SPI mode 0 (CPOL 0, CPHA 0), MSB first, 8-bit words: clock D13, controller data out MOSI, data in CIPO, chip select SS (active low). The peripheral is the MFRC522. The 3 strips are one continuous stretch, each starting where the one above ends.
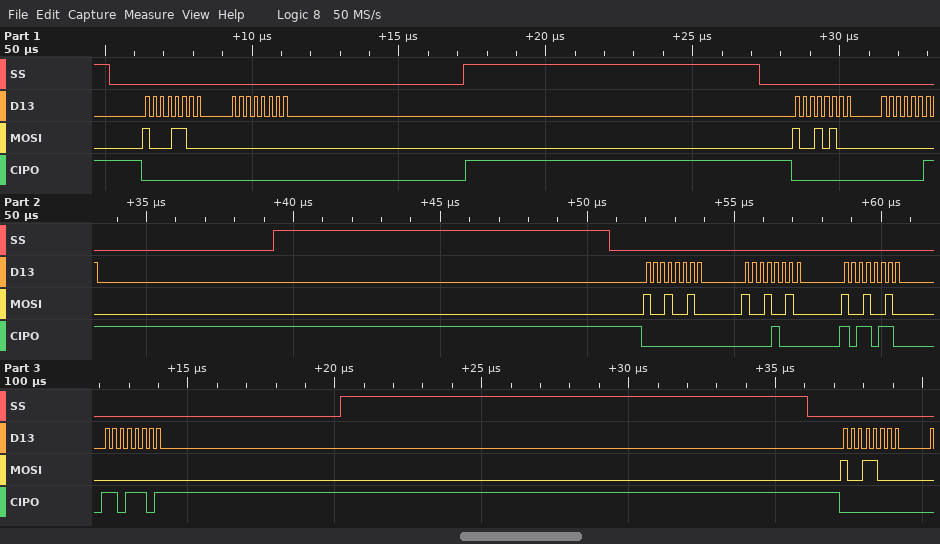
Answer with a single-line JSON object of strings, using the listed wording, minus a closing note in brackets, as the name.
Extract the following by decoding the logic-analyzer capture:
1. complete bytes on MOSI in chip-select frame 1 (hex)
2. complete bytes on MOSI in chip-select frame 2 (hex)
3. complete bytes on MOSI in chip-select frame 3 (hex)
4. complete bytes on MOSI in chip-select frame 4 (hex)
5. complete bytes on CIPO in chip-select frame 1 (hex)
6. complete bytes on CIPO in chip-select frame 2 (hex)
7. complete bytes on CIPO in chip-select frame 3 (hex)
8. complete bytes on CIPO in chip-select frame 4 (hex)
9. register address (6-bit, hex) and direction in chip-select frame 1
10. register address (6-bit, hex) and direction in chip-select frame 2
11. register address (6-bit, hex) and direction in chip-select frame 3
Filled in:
{"complete bytes on MOSI in chip-select frame 1": "0x8C 0x00", "complete bytes on MOSI in chip-select frame 2": "0x94 0x00", "complete bytes on MOSI in chip-select frame 3": "0x92 0x92 0x92 0x00", "complete bytes on MOSI in chip-select frame 4": "0x98", "complete bytes on CIPO in chip-select frame 1": "0x00 0x00", "complete bytes on CIPO in chip-select frame 2": "0x00 0x03", "complete bytes on CIPO in chip-select frame 3": "0x00 0x08 0xB6 0xDD", "complete bytes on CIPO in chip-select frame 4": "0x00", "register address (6-bit, hex) and direction in chip-select frame 1": "0x06 read", "register address (6-bit, hex) and direction in chip-select frame 2": "0x0A read", "register address (6-bit, hex) and direction in chip-select frame 3": "0x09 read"}
